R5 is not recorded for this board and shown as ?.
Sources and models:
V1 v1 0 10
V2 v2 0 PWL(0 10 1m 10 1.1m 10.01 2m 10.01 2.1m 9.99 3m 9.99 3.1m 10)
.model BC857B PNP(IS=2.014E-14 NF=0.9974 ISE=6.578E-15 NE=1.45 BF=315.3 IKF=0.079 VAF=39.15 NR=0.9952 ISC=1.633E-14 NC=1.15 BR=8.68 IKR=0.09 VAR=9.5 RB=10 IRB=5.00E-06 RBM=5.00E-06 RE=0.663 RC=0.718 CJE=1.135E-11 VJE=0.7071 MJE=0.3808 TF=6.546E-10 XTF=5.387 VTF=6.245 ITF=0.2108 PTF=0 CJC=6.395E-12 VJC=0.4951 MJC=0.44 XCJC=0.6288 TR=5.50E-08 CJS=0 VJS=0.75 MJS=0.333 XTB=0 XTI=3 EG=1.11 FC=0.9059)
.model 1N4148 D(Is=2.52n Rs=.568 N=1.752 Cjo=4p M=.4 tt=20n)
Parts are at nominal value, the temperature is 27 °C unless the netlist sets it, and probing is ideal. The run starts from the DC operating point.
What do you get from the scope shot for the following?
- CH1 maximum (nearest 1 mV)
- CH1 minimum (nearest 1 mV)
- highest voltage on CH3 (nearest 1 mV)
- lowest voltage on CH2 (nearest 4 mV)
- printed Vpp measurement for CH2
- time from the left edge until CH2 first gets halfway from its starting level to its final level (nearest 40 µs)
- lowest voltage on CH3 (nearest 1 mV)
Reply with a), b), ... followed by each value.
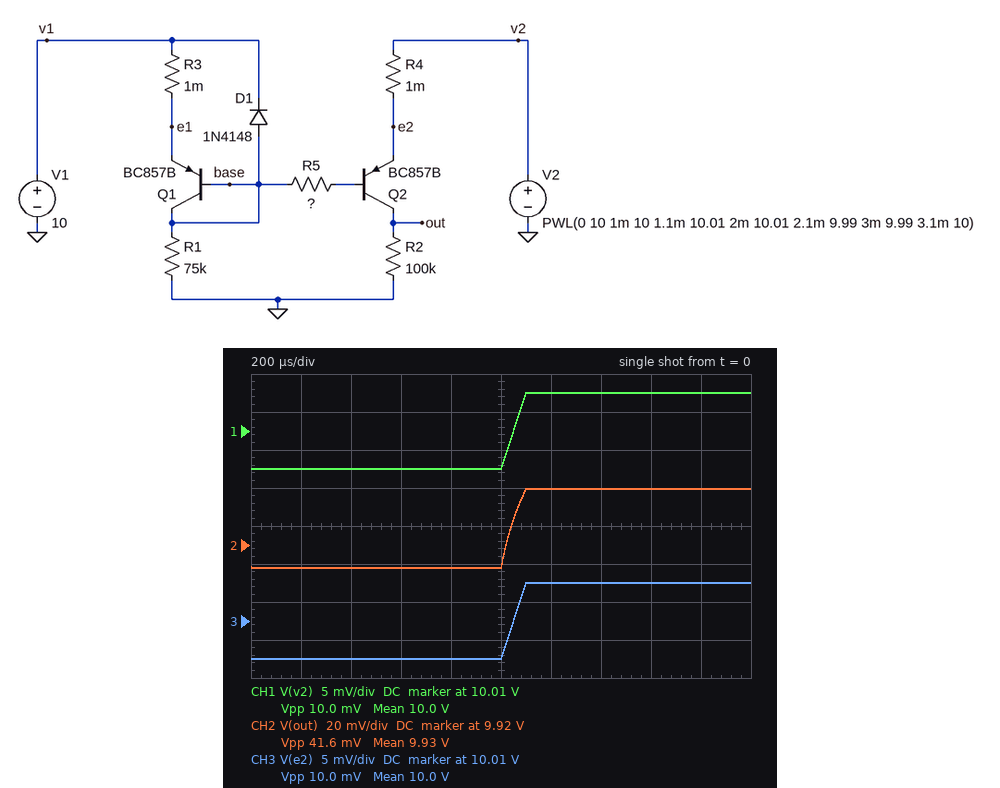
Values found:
a) 10.010 V
b) 10.000 V
c) 10.010 V
d) 9.908 V
e) 41.6 mV
f) 1.04 ms
g) 10.000 V
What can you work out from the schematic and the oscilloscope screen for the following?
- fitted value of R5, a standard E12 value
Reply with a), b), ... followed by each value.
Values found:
a) 4.7 kΩ
